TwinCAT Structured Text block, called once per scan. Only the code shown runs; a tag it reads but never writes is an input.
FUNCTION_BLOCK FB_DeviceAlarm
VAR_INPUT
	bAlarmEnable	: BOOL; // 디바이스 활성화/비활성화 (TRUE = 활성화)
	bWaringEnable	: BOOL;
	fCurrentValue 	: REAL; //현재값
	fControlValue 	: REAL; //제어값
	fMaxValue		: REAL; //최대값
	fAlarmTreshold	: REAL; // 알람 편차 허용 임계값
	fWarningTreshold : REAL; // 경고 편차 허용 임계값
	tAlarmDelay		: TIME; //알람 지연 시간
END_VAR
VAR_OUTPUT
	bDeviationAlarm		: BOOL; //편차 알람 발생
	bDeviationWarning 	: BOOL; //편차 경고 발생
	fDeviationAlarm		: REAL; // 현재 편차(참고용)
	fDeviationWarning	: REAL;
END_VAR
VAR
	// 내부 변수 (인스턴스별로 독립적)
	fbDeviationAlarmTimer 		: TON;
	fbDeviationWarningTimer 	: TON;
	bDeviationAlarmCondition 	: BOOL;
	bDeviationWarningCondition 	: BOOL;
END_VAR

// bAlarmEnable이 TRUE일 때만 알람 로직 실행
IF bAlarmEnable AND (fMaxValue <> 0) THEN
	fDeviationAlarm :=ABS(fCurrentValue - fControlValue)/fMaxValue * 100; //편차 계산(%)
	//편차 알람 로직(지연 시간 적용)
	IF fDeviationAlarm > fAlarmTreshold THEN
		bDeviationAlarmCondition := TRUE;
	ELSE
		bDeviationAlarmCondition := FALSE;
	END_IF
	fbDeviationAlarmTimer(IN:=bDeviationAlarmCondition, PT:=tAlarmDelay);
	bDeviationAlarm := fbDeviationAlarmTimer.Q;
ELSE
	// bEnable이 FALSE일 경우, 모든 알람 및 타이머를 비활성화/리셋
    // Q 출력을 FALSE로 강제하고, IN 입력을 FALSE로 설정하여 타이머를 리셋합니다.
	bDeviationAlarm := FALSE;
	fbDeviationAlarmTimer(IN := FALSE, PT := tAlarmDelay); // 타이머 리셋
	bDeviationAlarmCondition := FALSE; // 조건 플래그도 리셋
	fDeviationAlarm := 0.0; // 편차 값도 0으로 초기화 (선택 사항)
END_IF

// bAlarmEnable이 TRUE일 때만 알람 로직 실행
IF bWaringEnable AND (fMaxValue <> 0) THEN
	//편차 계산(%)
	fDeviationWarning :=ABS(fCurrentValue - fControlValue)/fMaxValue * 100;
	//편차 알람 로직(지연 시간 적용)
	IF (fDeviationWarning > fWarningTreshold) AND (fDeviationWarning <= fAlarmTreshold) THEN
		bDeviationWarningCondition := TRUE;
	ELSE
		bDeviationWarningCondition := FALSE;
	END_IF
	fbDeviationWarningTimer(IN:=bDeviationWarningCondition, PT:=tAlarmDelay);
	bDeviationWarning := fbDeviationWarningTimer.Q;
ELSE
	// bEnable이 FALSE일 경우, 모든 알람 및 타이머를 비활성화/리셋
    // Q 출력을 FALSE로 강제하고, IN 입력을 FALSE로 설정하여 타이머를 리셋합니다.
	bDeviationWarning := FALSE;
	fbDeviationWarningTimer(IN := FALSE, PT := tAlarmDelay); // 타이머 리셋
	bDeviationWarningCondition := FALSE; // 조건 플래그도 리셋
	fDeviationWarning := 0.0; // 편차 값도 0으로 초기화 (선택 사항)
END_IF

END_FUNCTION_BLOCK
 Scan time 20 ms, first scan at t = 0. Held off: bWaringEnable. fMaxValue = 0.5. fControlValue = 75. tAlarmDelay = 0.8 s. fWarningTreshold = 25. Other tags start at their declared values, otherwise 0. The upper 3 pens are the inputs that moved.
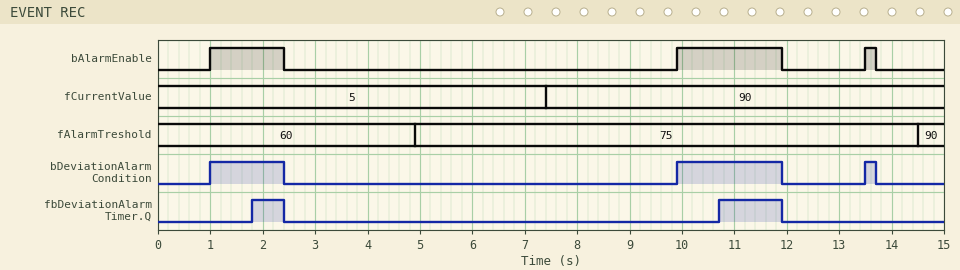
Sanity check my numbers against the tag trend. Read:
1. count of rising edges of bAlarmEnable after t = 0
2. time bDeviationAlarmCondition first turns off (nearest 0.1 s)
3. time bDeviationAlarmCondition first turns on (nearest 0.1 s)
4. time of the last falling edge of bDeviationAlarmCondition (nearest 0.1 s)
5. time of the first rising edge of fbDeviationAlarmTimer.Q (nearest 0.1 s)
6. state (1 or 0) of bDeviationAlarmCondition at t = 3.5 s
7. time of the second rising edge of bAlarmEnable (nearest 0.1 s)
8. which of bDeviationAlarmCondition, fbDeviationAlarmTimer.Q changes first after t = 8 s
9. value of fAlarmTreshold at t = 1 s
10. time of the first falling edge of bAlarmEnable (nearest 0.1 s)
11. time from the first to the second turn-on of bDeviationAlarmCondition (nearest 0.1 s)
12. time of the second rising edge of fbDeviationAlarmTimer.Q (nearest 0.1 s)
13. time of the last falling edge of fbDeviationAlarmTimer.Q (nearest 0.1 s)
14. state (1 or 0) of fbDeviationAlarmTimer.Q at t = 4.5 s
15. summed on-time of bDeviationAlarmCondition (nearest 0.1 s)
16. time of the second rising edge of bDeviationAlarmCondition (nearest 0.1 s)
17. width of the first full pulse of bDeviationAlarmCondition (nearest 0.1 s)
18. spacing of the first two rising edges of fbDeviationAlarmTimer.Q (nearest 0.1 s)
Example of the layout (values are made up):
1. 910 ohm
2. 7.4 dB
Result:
1. 3
2. 2.4 s
3. 1.0 s
4. 13.7 s
5. 1.8 s
6. 0
7. 9.9 s
8. bDeviationAlarmCondition
9. 60
10. 2.4 s
11. 8.9 s
12. 10.7 s
13. 11.9 s
14. 0
15. 3.6 s
16. 9.9 s
17. 1.4 s
18. 8.9 s
